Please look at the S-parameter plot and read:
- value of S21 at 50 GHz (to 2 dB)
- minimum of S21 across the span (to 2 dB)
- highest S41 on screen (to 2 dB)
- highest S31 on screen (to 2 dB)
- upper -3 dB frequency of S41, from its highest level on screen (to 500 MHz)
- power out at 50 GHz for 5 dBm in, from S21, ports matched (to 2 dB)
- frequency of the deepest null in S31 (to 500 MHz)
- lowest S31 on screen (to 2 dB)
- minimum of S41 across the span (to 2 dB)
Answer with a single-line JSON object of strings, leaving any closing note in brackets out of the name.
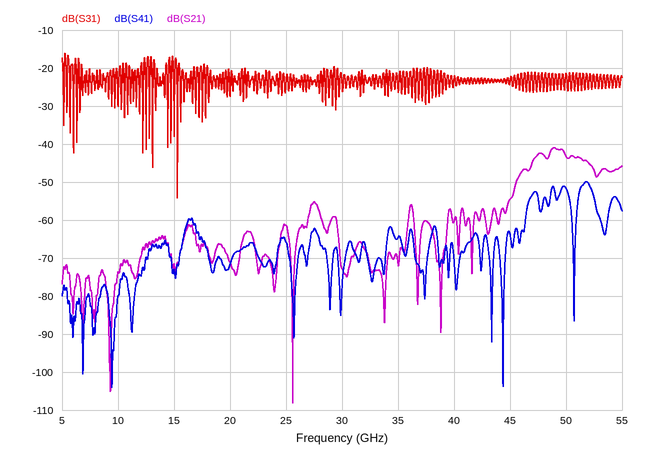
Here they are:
{"value of S21 at 50 GHz": "-44 dB", "minimum of S21 across the span": "-108 dB", "highest S41 on screen": "-50 dB", "highest S31 on screen": "-16 dB", "upper -3 dB frequency of S41, from its highest level on screen": "52.5 GHz", "power out at 50 GHz for 5 dBm in, from S21, ports matched": "-38 dBm", "frequency of the deepest null in S31": "15.5 GHz", "lowest S31 on screen": "-54 dB", "minimum of S41 across the span": "-104 dB"}
